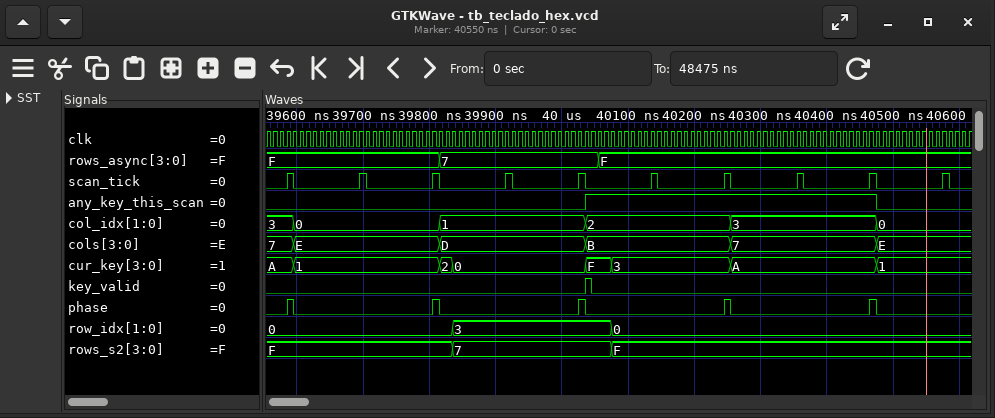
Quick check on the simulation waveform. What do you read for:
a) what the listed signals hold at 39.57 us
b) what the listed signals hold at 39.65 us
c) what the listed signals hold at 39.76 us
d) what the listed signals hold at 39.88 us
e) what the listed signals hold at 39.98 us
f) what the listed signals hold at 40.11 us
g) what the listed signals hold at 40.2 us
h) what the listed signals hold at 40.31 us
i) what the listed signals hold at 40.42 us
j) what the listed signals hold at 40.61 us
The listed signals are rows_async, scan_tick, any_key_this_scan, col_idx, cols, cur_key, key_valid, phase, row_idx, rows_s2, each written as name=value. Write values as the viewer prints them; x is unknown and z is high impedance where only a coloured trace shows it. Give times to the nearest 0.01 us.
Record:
rows_async=F, scan_tick=0, any_key_this_scan=0, col_idx=3, cols=7, cur_key=A, key_valid=0, phase=0, row_idx=0, rows_s2=F
rows_async=F, scan_tick=0, any_key_this_scan=0, col_idx=0, cols=E, cur_key=1, key_valid=0, phase=0, row_idx=0, rows_s2=F
rows_async=F, scan_tick=0, any_key_this_scan=0, col_idx=0, cols=E, cur_key=1, key_valid=0, phase=0, row_idx=0, rows_s2=F
rows_async=7, scan_tick=0, any_key_this_scan=0, col_idx=1, cols=D, cur_key=0, key_valid=0, phase=0, row_idx=3, rows_s2=7
rows_async=7, scan_tick=0, any_key_this_scan=0, col_idx=1, cols=D, cur_key=0, key_valid=0, phase=0, row_idx=3, rows_s2=7
rows_async=F, scan_tick=0, any_key_this_scan=1, col_idx=2, cols=B, cur_key=3, key_valid=0, phase=0, row_idx=0, rows_s2=F
rows_async=F, scan_tick=0, any_key_this_scan=1, col_idx=2, cols=B, cur_key=3, key_valid=0, phase=0, row_idx=0, rows_s2=F
rows_async=F, scan_tick=0, any_key_this_scan=1, col_idx=3, cols=7, cur_key=A, key_valid=0, phase=0, row_idx=0, rows_s2=F
rows_async=F, scan_tick=0, any_key_this_scan=1, col_idx=3, cols=7, cur_key=A, key_valid=0, phase=0, row_idx=0, rows_s2=F
rows_async=F, scan_tick=0, any_key_this_scan=0, col_idx=0, cols=E, cur_key=1, key_valid=0, phase=0, row_idx=0, rows_s2=F
